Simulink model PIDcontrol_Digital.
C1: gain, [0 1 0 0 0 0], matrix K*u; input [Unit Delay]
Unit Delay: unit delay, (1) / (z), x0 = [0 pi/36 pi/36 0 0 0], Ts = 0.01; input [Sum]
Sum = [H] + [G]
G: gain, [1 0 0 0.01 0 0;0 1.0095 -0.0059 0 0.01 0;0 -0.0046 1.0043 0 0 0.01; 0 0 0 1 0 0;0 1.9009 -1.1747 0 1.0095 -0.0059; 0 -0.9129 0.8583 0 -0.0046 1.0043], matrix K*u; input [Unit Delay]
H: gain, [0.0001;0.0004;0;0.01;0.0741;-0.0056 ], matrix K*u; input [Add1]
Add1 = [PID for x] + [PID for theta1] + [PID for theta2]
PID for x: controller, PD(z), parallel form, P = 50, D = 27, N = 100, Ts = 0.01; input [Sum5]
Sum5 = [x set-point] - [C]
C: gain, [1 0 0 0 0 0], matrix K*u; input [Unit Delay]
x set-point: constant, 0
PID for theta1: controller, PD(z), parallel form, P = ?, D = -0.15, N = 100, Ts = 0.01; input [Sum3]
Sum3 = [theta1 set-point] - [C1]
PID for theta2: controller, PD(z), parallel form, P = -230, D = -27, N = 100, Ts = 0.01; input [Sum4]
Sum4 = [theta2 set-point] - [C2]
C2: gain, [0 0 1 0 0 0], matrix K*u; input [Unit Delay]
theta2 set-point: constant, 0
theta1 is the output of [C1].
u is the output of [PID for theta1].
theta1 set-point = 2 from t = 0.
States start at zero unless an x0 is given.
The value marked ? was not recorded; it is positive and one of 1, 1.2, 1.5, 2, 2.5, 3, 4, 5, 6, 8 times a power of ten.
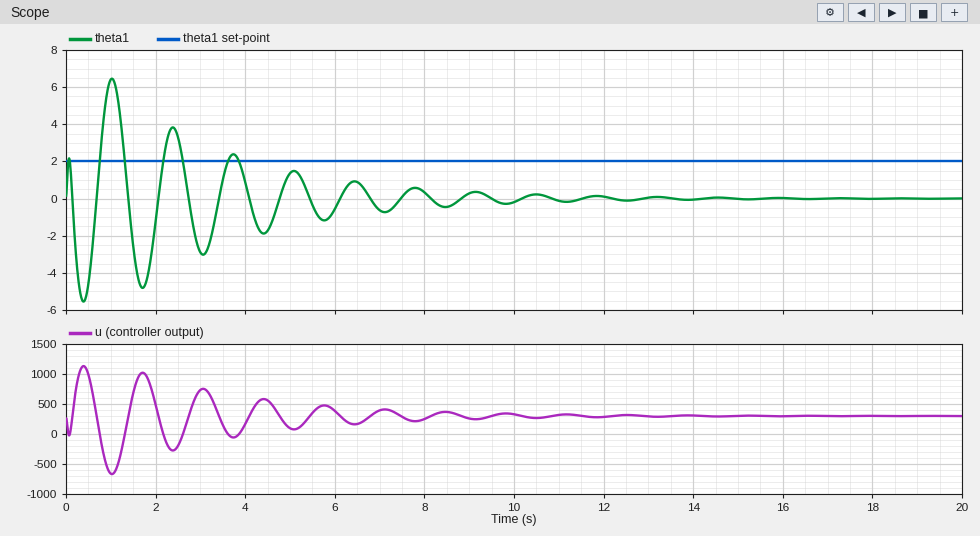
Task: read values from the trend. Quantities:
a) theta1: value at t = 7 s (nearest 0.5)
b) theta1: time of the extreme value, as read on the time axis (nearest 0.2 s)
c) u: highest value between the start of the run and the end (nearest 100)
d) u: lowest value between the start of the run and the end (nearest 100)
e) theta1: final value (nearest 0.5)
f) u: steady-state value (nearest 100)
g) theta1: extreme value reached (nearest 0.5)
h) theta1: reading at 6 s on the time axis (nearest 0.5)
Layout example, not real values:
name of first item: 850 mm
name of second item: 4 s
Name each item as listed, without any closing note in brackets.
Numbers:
theta1: value at t = 7 s: -0.5
theta1: time of the extreme value, as read on the time axis: 1.0 s
u: highest value between the start of the run and the end: 1100
u: lowest value between the start of the run and the end: -700
theta1: final value: 0.0
u: steady-state value: 300
theta1: extreme value reached: 6.5
theta1: reading at 6 s on the time axis: -0.5
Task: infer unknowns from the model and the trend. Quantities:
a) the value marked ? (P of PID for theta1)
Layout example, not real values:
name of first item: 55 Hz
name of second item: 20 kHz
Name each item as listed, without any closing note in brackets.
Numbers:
the value marked ?: 150
